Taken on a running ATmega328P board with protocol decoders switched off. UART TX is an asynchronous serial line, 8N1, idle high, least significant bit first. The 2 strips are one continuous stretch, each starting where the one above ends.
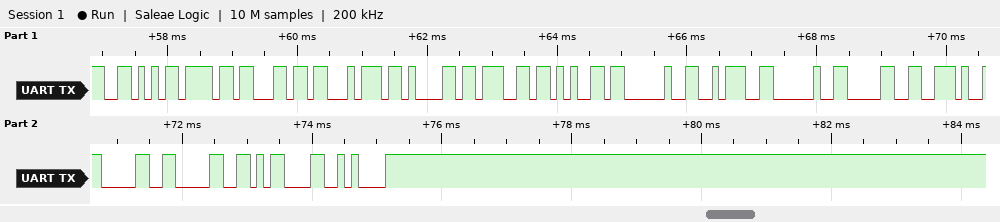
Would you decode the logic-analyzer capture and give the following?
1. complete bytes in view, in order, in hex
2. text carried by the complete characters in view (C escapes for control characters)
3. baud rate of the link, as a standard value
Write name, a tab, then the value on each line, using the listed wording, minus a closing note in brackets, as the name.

complete bytes in view, in order, in hex	0x56 0x6F 0x6C 0x74 0x61 0x67 0x65 0x20 0x3A 0x20 0x30 0x2E 0x30 0x30 0x0D 0x0A
text carried by the complete characters in view	"Voltage : 0.00\r\n"
baud rate of the link, as a standard value	9600 baud
